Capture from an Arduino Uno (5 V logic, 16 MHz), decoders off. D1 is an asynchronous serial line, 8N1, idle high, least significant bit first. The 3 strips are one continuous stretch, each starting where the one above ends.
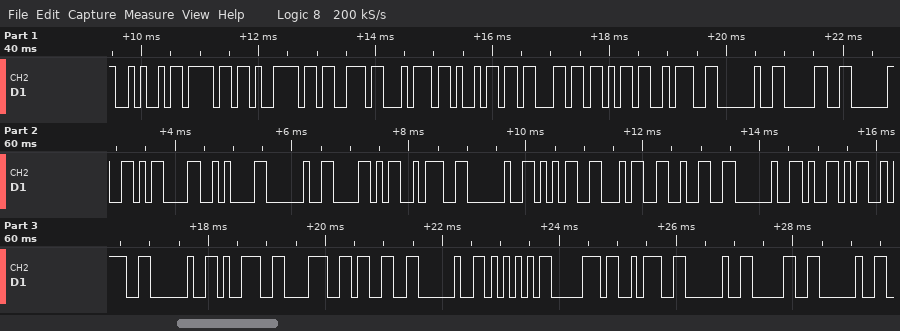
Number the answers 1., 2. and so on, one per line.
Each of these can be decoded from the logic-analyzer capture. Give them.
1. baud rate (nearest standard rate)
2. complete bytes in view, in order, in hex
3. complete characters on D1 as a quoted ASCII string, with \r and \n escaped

1. 9600 baud
2. 4A 6F 79 73 74 69 63 6B 3A 20 30 20 0D 0A 20 58 3A 20 35 34 32 20 59 3A 20 39 38 33 20 55 70 3A 20 30 20
3. "Joystick: 0 \r\n X: 542 Y: 983 Up: 0 "
